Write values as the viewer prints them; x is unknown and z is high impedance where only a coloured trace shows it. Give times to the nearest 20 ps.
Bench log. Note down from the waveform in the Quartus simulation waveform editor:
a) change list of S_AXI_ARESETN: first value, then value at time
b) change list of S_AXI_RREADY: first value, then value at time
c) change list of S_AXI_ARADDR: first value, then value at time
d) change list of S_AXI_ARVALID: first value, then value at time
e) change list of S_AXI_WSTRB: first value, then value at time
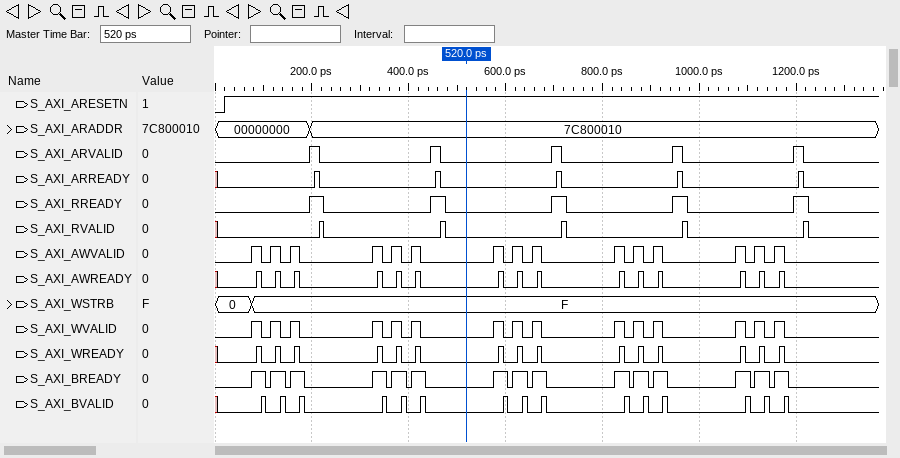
0, 1 at 20 ps
0, 1 at 200 ps, 0 at 220 ps, 1 at 440 ps, 0 at 480 ps, 1 at 700 ps, 0 at 720 ps, 1 at 940 ps, 0 at 980 ps, 1 at 1200 ps, 0 at 1220 ps
00000000, 7C800010 at 200 ps
0, 1 at 200 ps, 0 at 220 ps, 1 at 440 ps, 0 at 460 ps, 1 at 700 ps, 0 at 720 ps, 1 at 940 ps, 0 at 960 ps, 1 at 1200 ps, 0 at 1220 ps
0, F at 80 ps
